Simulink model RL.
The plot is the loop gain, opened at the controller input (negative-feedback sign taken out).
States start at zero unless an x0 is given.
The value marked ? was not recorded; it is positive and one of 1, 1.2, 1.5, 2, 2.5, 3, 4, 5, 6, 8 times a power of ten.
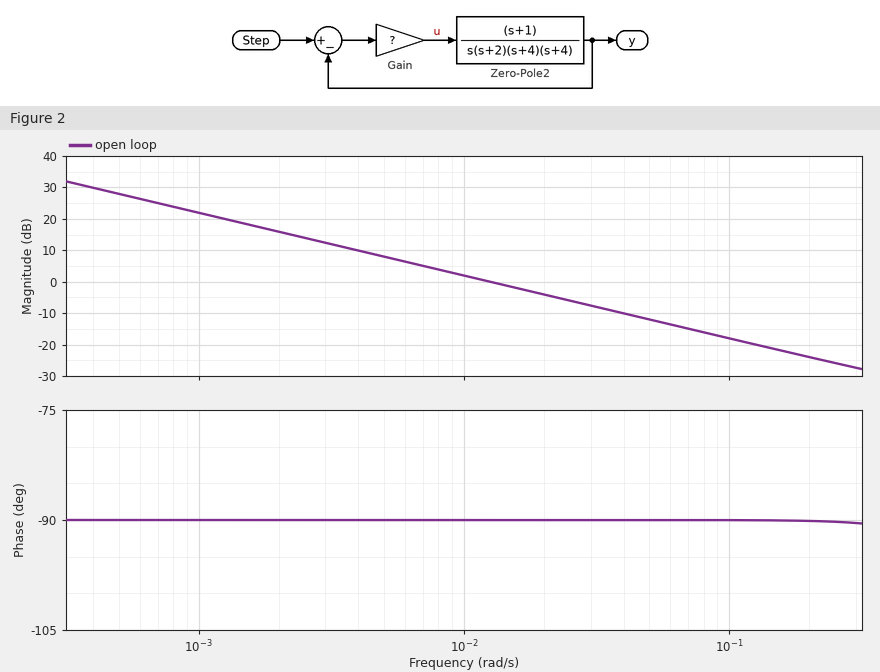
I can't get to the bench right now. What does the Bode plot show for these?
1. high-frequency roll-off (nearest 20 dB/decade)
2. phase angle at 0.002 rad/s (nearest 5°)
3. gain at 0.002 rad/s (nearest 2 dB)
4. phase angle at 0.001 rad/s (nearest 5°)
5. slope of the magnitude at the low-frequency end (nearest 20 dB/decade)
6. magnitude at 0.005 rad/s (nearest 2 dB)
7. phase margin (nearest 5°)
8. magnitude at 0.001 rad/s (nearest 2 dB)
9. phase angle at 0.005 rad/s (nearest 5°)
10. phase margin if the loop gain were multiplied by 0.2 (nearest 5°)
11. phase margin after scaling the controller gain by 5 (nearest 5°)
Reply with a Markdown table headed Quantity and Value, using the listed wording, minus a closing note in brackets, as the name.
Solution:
| Quantity | Value |
|---|---|
| high-frequency roll-off | -20 dB/decade |
| phase angle at 0.002 rad/s | -90° |
| gain at 0.002 rad/s | 16 dB |
| phase angle at 0.001 rad/s | -90° |
| slope of the magnitude at the low-frequency end | -20 dB/decade |
| magnitude at 0.005 rad/s | 8 dB |
| phase margin | 90° |
| magnitude at 0.001 rad/s | 22 dB |
| phase angle at 0.005 rad/s | -90° |
| phase margin if the loop gain were multiplied by 0.2 | 90° |
| phase margin after scaling the controller gain by 5 | 90° |
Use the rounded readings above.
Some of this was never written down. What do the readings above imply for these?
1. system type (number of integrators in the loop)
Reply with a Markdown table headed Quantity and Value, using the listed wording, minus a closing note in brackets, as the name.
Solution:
| Quantity | Value |
|---|---|
| system type | 1 |
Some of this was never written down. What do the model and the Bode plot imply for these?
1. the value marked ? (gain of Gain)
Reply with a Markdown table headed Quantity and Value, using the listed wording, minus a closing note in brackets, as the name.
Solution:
| Quantity | Value |
|---|---|
| the value marked ? | 0.4 |
